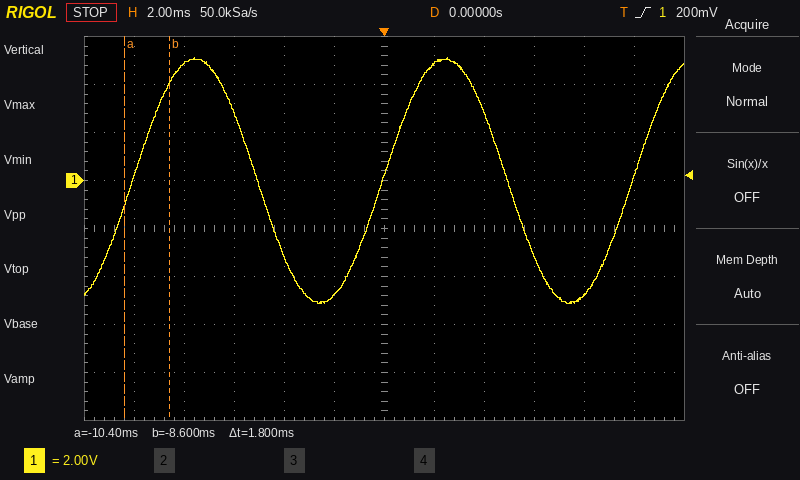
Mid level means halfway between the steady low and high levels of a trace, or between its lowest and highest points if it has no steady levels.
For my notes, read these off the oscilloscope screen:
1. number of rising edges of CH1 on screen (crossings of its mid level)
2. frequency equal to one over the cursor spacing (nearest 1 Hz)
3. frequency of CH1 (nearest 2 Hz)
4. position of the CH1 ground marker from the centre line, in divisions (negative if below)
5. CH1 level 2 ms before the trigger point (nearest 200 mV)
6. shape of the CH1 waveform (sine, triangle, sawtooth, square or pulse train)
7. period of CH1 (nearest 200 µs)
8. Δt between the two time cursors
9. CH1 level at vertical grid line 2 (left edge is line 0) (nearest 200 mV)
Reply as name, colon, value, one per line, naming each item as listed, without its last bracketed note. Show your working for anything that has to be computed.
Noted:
number of rising edges of CH1 on screen: 3
frequency equal to one over the cursor spacing: 1 / 1.8 ms ≈ 556 Hz
frequency of CH1: 1 / 10.0 ms ≈ 100 Hz
position of the CH1 ground marker from the centre line, in divisions: +1.0 div
CH1 level 2 ms before the trigger point: -4.8 V
shape of the CH1 waveform: sine
period of CH1: 10.0 ms
Δt between the two time cursors: 1.8 ms
CH1 level at vertical grid line 2 (left edge is line 0): 4.8 V
